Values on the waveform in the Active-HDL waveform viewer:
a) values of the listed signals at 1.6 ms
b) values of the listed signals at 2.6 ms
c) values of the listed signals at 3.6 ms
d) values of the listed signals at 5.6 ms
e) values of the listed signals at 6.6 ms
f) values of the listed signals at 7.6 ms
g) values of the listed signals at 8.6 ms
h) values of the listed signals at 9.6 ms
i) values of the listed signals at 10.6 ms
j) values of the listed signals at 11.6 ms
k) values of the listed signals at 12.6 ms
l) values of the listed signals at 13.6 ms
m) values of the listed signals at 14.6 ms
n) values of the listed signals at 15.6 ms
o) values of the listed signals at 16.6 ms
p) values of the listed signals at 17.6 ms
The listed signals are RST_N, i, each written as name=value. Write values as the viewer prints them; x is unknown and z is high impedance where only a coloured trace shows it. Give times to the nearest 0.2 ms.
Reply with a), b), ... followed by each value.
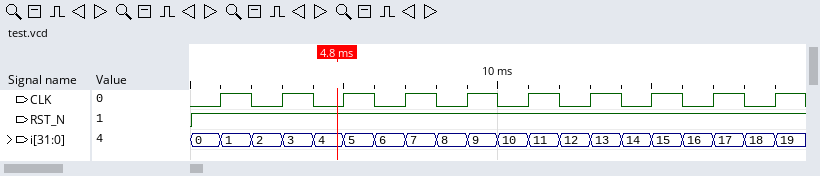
a) RST_N=1, i=1
b) RST_N=1, i=2
c) RST_N=1, i=3
d) RST_N=1, i=5
e) RST_N=1, i=6
f) RST_N=1, i=7
g) RST_N=1, i=8
h) RST_N=1, i=9
i) RST_N=1, i=10
j) RST_N=1, i=11
k) RST_N=1, i=12
l) RST_N=1, i=13
m) RST_N=1, i=14
n) RST_N=1, i=15
o) RST_N=1, i=16
p) RST_N=1, i=17
